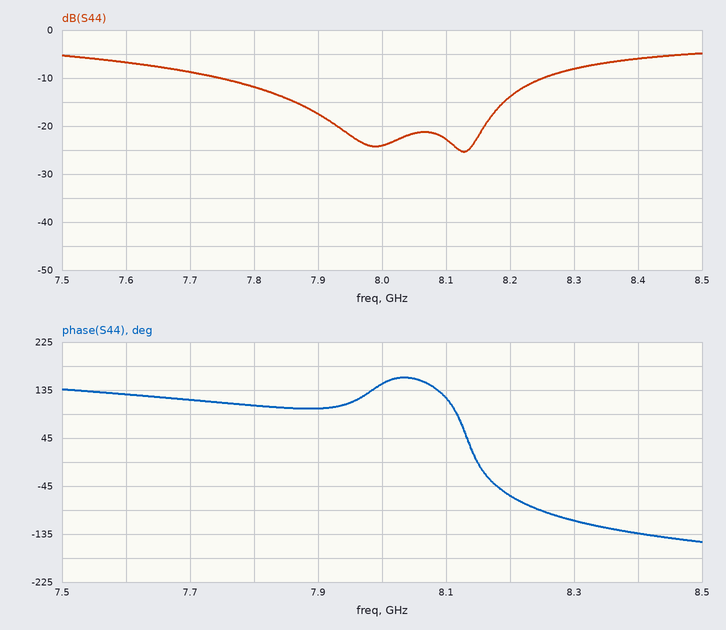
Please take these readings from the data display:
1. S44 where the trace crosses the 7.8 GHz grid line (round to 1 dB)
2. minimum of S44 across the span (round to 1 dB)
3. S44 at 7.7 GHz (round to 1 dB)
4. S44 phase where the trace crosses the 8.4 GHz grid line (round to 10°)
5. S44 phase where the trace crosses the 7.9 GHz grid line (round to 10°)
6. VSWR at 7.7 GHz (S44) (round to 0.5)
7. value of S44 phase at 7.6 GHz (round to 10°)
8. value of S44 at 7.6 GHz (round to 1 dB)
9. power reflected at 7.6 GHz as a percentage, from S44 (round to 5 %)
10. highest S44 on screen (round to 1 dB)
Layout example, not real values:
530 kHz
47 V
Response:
-12 dB
-25 dB
-9 dB
-130°
100°
2.0
130°
-7 dB
20 %
-5 dB
